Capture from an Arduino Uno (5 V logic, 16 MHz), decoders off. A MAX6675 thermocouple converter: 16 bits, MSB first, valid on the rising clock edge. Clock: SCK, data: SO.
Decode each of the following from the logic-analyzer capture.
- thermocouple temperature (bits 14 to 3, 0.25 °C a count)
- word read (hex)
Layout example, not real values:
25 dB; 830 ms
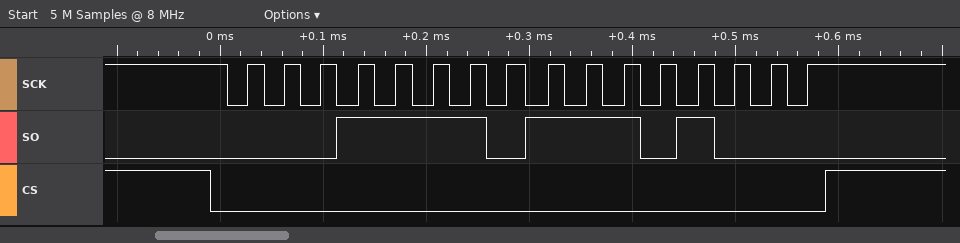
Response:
247.25 °C; 0x1EE8
